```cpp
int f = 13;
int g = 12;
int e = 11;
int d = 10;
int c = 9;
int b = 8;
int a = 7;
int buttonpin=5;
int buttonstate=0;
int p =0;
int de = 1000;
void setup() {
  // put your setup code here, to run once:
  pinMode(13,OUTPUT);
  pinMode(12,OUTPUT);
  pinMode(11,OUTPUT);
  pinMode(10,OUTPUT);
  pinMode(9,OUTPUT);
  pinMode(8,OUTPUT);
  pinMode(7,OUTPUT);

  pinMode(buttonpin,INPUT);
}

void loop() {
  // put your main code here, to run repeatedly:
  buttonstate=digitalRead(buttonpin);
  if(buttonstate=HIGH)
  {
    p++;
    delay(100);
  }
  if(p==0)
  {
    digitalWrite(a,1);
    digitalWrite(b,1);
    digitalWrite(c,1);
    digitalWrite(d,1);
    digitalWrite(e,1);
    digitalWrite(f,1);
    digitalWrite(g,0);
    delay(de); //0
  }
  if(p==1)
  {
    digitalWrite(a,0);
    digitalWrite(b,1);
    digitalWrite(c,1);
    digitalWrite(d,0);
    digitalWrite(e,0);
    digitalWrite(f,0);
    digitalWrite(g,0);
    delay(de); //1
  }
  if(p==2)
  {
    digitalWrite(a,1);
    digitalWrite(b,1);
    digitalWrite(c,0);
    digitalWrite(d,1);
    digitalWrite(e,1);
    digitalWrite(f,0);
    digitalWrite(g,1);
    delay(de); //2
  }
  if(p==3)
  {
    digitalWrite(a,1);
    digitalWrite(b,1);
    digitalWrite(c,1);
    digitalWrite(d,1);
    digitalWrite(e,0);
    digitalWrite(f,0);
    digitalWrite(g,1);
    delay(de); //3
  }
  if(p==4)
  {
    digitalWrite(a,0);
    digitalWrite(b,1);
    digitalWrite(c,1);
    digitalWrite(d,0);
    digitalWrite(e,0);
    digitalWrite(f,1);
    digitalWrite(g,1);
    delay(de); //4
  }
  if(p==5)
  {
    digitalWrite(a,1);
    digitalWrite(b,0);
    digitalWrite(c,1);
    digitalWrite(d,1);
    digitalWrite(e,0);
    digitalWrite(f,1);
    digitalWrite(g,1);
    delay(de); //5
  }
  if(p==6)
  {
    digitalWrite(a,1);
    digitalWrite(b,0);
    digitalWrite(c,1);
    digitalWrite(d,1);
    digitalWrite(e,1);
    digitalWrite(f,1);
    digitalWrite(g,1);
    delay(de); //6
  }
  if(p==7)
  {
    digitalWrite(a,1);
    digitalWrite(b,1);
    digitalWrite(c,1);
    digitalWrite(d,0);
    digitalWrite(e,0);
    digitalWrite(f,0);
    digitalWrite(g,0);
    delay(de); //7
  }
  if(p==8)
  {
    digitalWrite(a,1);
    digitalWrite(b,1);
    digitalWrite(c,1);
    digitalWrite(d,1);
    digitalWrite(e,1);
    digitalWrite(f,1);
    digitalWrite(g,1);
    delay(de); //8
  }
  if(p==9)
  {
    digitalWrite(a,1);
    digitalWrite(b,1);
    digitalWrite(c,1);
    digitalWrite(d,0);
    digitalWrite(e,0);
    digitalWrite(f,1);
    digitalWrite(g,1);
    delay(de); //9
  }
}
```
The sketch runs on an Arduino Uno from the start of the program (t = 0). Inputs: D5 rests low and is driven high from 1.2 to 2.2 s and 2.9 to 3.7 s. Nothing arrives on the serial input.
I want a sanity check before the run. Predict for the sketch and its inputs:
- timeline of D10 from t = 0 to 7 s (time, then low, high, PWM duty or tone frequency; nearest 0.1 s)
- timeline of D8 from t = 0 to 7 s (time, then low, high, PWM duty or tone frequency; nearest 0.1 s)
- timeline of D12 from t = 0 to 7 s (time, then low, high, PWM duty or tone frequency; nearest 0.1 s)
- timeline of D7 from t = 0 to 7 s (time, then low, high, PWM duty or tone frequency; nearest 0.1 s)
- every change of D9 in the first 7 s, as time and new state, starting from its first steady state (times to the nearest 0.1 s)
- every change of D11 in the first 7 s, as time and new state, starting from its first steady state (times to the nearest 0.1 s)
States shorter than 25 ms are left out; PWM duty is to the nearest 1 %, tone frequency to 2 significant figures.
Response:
0 s low; 1.2 s high; 3.4 s low; 4.5 s high; 6.7 s low
0 s low; 0.1 s high; 4.5 s low; 6.7 s high
0 s low; 1.2 s high; 6.7 s low
0 s low; 1.2 s high; 3.4 s low; 4.5 s high
0 s low; 0.1 s high; 1.2 s low; 2.3 s high
0 s low; 1.2 s high; 2.3 s low; 5.6 s high; 6.7 s low
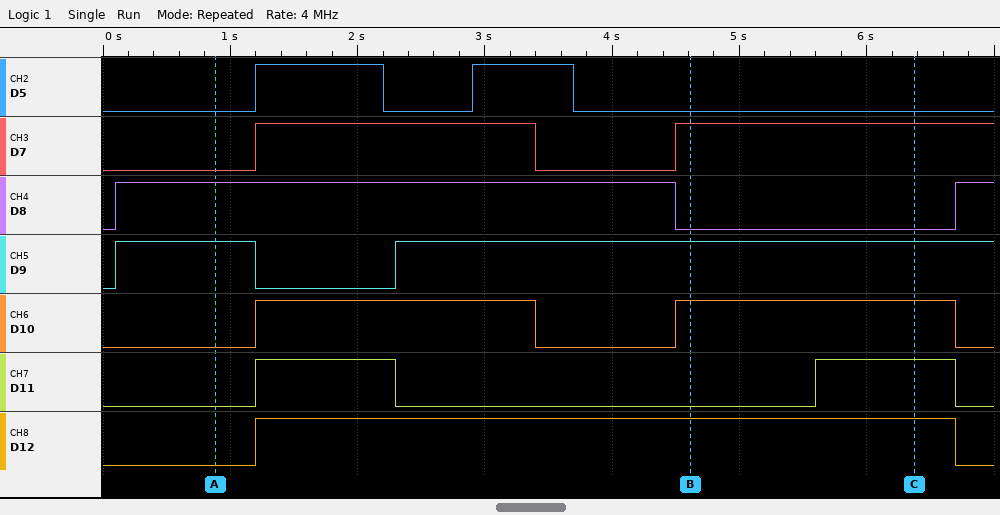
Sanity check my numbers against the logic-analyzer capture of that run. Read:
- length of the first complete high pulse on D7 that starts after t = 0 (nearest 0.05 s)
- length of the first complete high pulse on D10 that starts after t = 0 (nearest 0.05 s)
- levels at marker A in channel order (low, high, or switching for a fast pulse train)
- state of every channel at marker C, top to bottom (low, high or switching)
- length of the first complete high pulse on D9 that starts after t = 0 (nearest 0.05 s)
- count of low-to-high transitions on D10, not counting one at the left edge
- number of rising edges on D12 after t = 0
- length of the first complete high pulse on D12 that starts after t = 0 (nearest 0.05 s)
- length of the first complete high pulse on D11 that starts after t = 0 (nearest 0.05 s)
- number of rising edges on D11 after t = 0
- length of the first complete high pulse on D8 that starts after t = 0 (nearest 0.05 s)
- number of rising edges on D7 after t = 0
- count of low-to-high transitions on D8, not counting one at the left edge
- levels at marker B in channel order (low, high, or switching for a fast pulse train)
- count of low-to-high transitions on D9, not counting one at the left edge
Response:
2.20 s
2.20 s
D5 low, D7 low, D8 high, D9 high, D10 low, D11 low, D12 low
D5 low, D7 high, D8 low, D9 high, D10 high, D11 high, D12 high
1.10 s
2
1
5.50 s
1.10 s
2
4.40 s
2
2
D5 low, D7 high, D8 low, D9 high, D10 high, D11 low, D12 high
2
